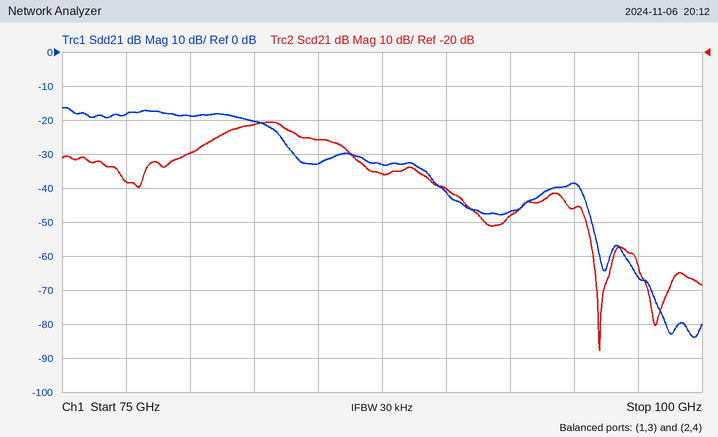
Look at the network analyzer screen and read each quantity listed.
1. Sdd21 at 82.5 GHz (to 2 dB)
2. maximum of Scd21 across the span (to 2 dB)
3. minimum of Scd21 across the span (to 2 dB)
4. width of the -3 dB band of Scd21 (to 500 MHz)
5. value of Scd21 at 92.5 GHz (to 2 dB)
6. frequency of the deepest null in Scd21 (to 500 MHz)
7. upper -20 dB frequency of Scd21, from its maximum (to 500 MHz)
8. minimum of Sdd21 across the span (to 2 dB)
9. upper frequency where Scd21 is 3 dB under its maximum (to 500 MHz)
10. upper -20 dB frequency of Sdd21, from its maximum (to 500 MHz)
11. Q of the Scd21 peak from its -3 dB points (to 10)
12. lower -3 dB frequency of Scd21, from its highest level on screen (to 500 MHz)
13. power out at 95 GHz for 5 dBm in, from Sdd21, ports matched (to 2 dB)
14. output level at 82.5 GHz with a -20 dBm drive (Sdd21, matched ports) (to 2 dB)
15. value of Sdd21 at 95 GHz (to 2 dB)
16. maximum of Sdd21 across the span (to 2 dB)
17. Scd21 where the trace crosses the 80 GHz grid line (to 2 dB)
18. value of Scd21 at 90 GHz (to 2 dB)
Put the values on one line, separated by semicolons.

-20 dB; -40 dB; -108 dB; 2.5 GHz; -68 dB; 96.0 GHz; 90.0 GHz; -84 dB; 84.0 GHz; 89.5 GHz; 30; 81.5 GHz; -34 dBm; -40 dBm; -38 dB; -16 dB; -50 dB; -60 dB
